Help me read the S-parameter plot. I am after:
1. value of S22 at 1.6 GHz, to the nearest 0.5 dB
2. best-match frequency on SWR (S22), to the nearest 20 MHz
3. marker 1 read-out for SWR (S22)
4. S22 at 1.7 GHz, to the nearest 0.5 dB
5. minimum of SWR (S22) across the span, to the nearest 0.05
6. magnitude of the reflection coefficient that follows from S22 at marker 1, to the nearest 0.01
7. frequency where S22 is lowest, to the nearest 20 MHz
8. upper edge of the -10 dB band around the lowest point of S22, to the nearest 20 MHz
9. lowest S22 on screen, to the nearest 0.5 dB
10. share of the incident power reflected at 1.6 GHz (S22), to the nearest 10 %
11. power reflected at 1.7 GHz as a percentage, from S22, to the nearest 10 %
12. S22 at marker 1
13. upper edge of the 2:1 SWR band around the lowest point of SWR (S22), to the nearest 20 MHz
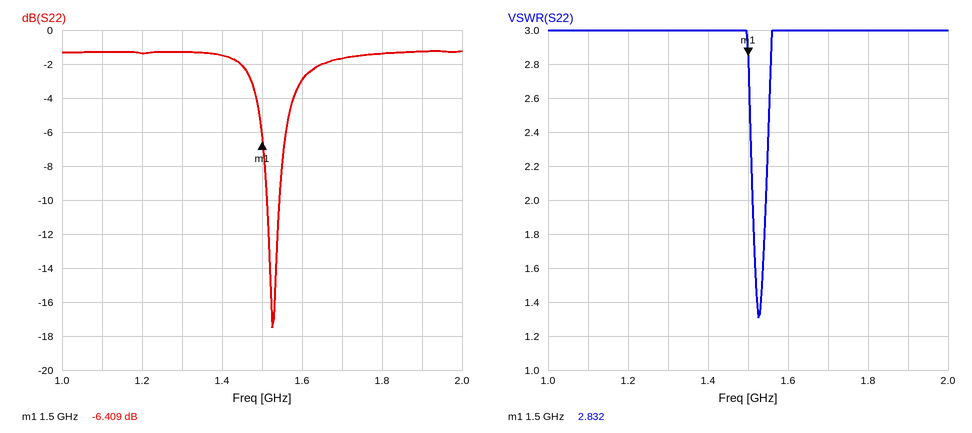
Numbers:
-3.0 dB
1.52 GHz
2.832
-1.5 dB
1.30
0.48
1.52 GHz
1.54 GHz
-17.5 dB
50 %
70 %
-6.409 dB
1.54 GHz
